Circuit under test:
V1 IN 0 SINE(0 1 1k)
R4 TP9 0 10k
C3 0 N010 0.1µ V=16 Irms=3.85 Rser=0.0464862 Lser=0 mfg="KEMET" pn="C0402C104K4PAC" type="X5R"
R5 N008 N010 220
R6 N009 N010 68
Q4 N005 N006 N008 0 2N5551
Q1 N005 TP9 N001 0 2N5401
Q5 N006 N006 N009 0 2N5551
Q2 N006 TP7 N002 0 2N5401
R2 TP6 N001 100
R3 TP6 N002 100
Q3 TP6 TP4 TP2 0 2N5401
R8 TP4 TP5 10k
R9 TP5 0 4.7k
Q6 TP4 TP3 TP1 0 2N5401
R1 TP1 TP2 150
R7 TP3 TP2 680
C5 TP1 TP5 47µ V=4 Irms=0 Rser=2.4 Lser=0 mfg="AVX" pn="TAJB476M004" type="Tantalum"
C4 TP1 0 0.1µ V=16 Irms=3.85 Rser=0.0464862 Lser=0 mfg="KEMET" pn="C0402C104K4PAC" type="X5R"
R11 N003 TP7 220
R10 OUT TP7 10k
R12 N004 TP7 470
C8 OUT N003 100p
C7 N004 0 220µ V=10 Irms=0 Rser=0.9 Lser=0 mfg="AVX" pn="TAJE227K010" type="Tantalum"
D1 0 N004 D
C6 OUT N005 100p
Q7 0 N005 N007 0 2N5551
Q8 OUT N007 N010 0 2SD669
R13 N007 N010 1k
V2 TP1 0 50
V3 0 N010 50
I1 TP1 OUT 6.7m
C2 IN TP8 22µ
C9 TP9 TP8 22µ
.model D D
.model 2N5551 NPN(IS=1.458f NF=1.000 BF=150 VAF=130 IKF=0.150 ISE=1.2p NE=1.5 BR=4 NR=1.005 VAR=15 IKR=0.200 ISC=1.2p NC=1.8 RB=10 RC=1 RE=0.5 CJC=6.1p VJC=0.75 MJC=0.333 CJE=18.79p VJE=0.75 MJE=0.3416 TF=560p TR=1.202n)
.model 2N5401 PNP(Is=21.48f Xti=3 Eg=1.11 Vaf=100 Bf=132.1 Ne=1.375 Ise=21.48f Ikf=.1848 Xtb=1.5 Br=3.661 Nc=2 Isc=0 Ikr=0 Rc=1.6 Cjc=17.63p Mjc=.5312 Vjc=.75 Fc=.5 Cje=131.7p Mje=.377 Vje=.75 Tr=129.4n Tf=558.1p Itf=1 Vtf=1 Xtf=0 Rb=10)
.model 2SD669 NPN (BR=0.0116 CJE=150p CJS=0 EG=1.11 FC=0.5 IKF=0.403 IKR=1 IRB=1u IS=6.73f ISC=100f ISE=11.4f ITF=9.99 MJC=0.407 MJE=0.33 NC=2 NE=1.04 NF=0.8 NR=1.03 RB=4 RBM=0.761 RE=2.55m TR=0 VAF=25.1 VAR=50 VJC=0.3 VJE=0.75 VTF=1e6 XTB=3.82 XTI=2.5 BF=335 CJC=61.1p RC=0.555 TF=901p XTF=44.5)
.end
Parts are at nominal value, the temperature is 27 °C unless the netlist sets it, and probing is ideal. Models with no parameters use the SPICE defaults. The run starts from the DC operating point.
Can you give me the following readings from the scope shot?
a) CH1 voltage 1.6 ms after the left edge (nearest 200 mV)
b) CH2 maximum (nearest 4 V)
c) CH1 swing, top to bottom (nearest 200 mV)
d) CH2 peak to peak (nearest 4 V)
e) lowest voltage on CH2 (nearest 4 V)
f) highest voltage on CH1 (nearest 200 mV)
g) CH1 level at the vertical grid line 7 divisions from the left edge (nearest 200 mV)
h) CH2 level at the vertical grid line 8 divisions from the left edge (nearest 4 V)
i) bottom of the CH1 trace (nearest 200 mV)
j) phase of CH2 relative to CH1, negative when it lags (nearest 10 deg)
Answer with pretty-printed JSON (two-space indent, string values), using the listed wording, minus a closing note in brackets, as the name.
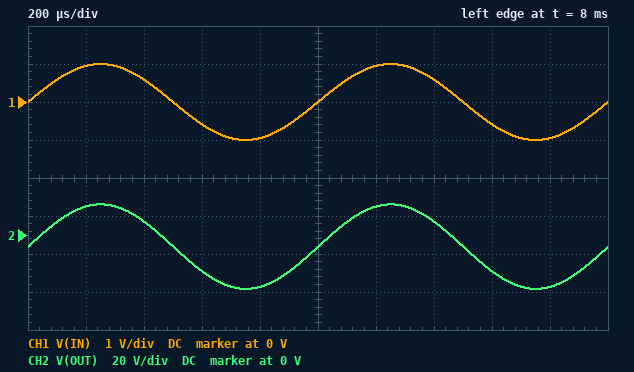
{
  "CH1 voltage 1.6 ms after the left edge": "-600 mV",
  "CH2 maximum": "16 V",
  "CH1 swing, top to bottom": "2.0 V",
  "CH2 peak to peak": "44 V",
  "lowest voltage on CH2": "-28 V",
  "highest voltage on CH1": "1.0 V",
  "CH1 level at the vertical grid line 7 divisions from the left edge": "600 mV",
  "CH2 level at the vertical grid line 8 divisions from the left edge": "-20 V",
  "bottom of the CH1 trace": "-1.0 V",
  "phase of CH2 relative to CH1, negative when it lags": "0 deg"
}
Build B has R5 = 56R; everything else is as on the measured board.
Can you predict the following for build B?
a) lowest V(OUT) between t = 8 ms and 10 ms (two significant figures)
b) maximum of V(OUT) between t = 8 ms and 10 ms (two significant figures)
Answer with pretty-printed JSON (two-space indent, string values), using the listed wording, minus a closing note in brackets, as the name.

{
  "lowest V(OUT) between t = 8 ms and 10 ms": "-24 V",
  "maximum of V(OUT) between t = 8 ms and 10 ms": "21 V"
}
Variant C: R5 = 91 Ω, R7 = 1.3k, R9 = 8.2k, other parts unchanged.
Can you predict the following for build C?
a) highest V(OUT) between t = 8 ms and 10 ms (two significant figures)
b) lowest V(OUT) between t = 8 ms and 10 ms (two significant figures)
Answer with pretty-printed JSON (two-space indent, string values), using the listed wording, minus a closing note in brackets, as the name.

{
  "highest V(OUT) between t = 8 ms and 10 ms": "19 V",
  "lowest V(OUT) between t = 8 ms and 10 ms": "-26 V"
}
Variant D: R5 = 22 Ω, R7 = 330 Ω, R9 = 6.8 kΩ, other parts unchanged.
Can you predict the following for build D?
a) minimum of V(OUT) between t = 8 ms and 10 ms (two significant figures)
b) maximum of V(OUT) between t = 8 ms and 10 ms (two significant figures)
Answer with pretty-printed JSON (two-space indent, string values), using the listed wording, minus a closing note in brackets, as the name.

{
  "minimum of V(OUT) between t = 8 ms and 10 ms": "-22 V",
  "maximum of V(OUT) between t = 8 ms and 10 ms": "22 V"
}
